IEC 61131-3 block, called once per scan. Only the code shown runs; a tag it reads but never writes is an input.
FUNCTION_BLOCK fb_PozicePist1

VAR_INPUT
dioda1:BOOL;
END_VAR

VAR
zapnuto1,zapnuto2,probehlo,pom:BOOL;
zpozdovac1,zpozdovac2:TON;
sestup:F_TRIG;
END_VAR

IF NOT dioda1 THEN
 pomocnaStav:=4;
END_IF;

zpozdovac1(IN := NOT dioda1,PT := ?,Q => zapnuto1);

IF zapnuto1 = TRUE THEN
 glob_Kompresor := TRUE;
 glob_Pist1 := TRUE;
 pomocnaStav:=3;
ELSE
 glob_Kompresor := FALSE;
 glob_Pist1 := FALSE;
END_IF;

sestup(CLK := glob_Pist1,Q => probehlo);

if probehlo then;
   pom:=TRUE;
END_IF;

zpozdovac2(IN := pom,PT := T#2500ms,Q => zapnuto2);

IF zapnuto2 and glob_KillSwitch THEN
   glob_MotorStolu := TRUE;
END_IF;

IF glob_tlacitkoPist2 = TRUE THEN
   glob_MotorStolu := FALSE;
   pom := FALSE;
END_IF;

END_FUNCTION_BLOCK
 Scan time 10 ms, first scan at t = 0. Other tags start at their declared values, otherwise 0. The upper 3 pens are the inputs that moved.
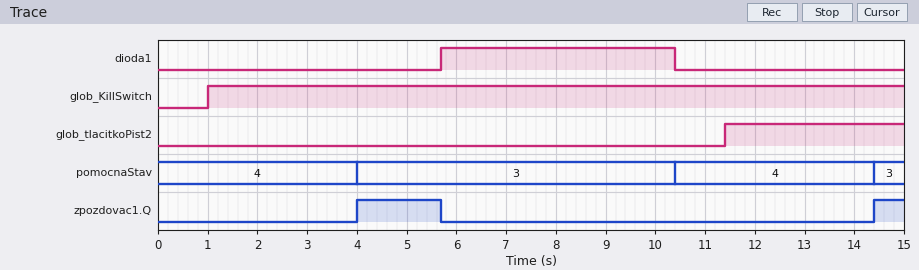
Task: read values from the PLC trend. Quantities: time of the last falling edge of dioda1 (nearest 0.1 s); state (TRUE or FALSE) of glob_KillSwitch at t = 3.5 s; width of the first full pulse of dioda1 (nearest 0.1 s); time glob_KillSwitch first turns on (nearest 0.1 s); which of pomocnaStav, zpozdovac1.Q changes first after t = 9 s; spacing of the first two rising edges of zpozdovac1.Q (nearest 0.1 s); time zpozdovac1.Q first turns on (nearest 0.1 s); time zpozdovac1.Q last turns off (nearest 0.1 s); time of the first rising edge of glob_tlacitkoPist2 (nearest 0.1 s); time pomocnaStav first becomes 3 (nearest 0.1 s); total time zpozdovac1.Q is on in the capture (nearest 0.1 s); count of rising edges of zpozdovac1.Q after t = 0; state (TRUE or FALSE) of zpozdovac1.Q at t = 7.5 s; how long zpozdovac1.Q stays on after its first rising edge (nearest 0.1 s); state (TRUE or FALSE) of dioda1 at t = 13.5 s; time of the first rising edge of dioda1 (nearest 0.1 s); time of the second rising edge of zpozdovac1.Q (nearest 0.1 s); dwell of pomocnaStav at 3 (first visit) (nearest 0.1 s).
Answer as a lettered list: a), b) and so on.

a) 10.4 s
b) TRUE
c) 4.7 s
d) 1.0 s
e) pomocnaStav
f) 10.4 s
g) 4.0 s
h) 5.7 s
i) 11.4 s
j) 4.0 s
k) 2.3 s
l) 2
m) FALSE
n) 1.7 s
o) FALSE
p) 5.7 s
q) 14.4 s
r) 6.4 s
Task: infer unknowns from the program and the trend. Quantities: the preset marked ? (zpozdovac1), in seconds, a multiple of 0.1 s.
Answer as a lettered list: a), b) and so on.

a) 4.0 s
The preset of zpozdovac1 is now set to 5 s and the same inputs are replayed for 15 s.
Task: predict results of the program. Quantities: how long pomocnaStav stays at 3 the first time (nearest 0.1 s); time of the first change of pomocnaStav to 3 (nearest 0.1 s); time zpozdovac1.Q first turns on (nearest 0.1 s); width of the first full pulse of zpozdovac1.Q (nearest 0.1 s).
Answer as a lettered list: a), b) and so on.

a) 5.4 s
b) 5.0 s
c) 5.0 s
d) 0.7 s
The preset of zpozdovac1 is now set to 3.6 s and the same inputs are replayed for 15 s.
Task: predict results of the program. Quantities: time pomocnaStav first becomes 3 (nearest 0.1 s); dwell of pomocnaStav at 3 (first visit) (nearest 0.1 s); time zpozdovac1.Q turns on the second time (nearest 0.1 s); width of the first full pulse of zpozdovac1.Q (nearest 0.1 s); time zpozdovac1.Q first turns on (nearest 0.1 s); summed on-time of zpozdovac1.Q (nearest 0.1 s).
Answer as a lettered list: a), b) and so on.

a) 3.6 s
b) 6.8 s
c) 14.0 s
d) 2.1 s
e) 3.6 s
f) 3.1 s
